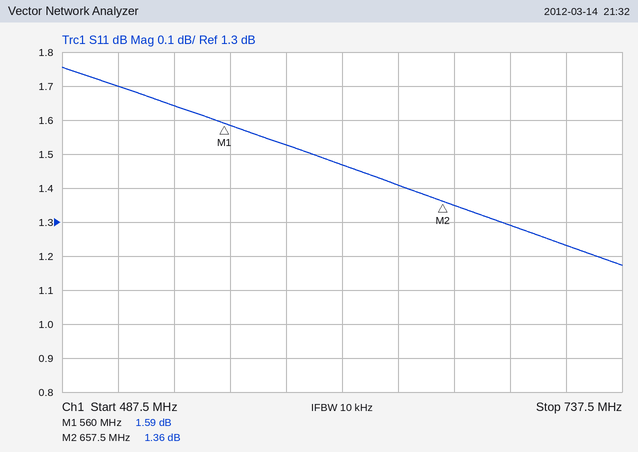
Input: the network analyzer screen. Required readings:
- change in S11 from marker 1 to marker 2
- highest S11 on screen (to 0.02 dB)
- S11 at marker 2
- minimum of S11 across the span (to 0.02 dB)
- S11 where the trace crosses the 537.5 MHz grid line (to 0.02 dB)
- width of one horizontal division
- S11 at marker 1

-0.23 dB
1.76 dB
1.36 dB
1.18 dB
1.64 dB
25 MHz
1.59 dB
